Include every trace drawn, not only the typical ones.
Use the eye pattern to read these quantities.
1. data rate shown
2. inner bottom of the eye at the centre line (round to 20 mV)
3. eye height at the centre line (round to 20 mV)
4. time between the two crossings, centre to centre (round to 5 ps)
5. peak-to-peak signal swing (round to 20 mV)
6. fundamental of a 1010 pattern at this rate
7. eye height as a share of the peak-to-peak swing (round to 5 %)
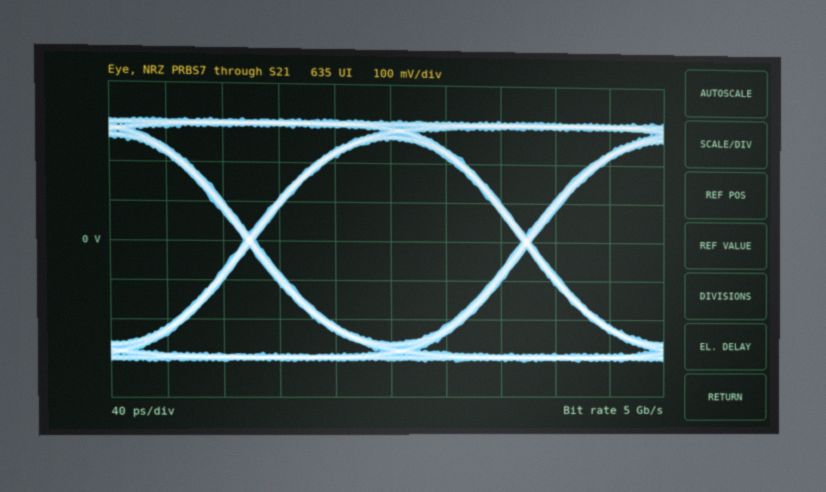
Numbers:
5 Gb/s
-260 mV
520 mV
200 ps
620 mV
2.5 GHz
85 %
